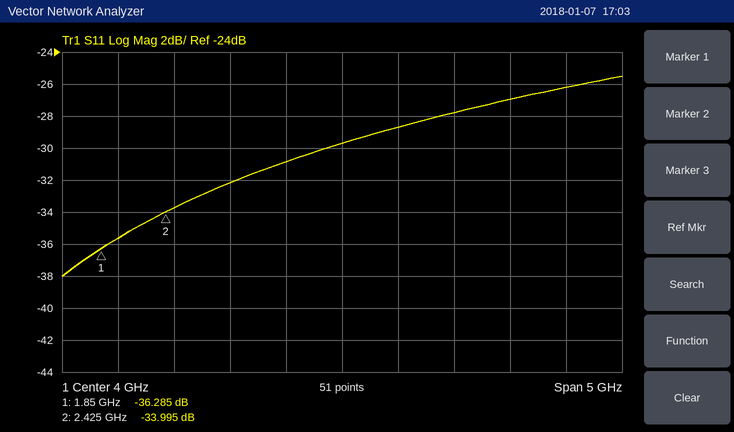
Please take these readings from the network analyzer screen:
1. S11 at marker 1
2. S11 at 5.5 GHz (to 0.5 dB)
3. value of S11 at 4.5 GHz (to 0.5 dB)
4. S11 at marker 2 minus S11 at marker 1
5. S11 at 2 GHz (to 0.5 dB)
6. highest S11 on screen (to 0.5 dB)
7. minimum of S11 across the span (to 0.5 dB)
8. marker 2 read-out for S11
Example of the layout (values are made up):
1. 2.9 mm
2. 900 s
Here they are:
1. -36.285 dB
2. -27.0 dB
3. -28.5 dB
4. 2.290 dB
5. -35.5 dB
6. -25.5 dB
7. -38.0 dB
8. -33.995 dB
